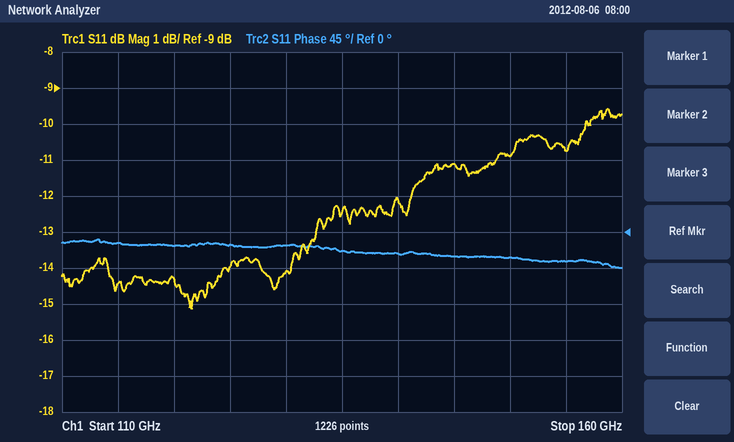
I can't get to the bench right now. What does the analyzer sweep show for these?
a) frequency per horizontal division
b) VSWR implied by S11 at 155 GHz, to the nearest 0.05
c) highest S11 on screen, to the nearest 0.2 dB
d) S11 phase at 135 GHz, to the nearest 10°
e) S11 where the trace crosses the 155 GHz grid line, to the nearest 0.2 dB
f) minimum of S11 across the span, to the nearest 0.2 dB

5 GHz
1.80
-9.6 dB
-20°
-10.8 dB
-15.2 dB
